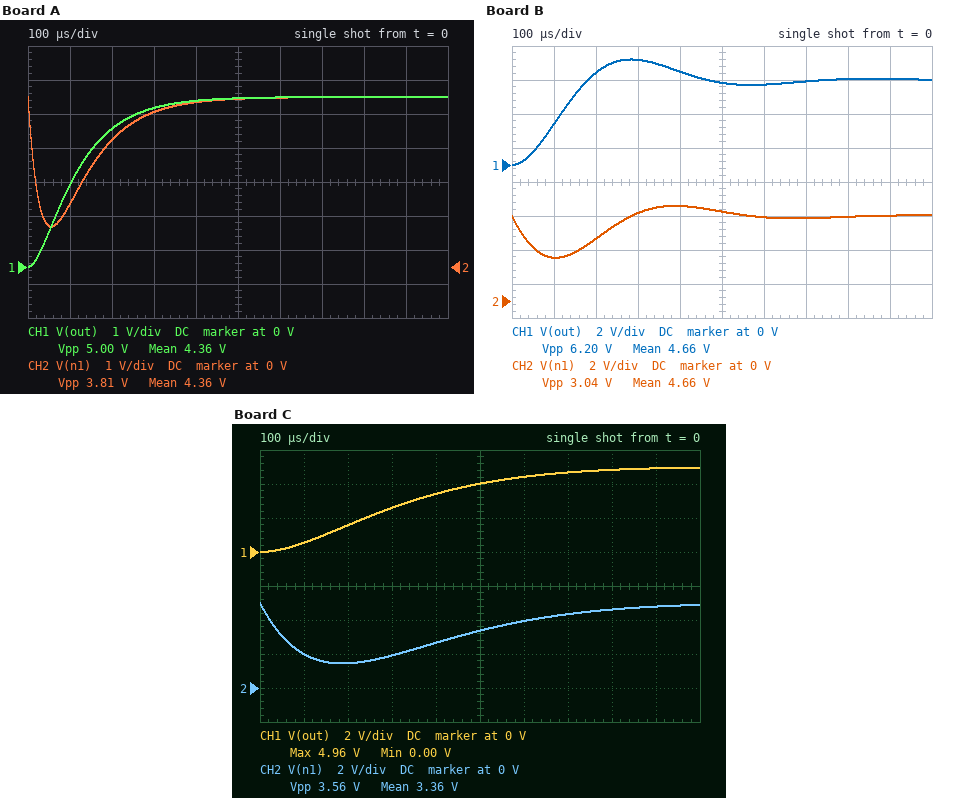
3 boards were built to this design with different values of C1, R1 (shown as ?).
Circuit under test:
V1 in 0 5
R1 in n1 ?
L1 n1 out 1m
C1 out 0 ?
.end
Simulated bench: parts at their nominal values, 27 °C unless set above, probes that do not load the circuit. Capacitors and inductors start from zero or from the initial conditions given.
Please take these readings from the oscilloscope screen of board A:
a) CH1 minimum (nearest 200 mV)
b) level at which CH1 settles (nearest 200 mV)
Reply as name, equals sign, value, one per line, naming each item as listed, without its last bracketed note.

CH1 minimum = 0 V
level at which CH1 settles = 5.0 V
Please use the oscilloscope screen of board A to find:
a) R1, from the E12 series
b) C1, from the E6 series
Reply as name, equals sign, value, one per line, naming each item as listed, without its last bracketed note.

R1, from the E12 series = 39 Ω
C1, from the E6 series = 3.3 µF
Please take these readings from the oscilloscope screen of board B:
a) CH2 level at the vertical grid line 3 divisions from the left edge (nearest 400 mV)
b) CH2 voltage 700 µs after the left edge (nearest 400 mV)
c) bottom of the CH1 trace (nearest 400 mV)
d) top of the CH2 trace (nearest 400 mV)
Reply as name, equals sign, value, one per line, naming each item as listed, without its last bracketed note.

CH2 level at the vertical grid line 3 divisions from the left edge = 5.2 V
CH2 voltage 700 µs after the left edge = 4.8 V
bottom of the CH1 trace = 0 V
top of the CH2 trace = 5.6 V
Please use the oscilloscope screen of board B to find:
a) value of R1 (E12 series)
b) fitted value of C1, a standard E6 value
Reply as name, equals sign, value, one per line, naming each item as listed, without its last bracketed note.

value of R1 = 10 Ω
fitted value of C1, a standard E6 value = 6.8 µF
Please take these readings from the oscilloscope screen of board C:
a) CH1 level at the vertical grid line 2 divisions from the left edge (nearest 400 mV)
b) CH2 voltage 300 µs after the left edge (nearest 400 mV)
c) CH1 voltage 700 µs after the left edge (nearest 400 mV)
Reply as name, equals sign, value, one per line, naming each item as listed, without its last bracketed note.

CH1 level at the vertical grid line 2 divisions from the left edge = 1.6 V
CH2 voltage 300 µs after the left edge = 2.0 V
CH1 voltage 700 µs after the left edge = 4.8 V
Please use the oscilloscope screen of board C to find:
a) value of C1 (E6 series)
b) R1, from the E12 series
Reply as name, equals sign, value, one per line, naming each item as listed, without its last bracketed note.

value of C1 = 33 µF
R1, from the E12 series = 10 Ω
